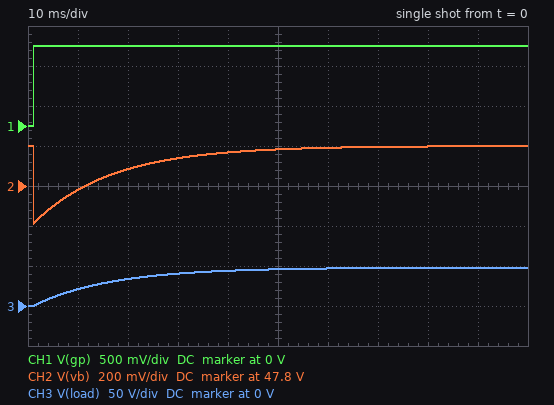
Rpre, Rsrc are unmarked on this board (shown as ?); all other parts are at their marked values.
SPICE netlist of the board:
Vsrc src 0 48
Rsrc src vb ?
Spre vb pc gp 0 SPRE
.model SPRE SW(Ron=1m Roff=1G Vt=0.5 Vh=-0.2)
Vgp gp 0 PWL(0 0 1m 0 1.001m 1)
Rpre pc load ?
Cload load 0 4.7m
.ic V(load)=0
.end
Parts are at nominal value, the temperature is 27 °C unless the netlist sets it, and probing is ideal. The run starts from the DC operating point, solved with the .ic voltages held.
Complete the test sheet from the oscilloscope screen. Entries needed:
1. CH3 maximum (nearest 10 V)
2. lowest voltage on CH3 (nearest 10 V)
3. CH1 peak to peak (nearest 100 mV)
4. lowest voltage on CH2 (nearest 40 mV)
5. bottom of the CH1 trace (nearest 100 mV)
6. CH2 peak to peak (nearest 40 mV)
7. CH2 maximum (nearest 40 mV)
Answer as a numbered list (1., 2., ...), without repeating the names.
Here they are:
1. 50 V
2. 0 V
3. 1.0 V
4. 47.60 V
5. 0 V
6. 400 mV
7. 48.00 V
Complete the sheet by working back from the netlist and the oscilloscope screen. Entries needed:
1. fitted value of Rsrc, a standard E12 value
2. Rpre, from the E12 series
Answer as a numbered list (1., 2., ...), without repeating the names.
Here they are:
1. 0.027 Ω
2. 3.3 Ω
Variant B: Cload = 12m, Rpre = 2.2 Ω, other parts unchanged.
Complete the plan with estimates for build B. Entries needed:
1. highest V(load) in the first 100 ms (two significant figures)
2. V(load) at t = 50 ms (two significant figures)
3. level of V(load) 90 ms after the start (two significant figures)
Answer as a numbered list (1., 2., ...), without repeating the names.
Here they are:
1. 47 V
2. 40 V
3. 46 V
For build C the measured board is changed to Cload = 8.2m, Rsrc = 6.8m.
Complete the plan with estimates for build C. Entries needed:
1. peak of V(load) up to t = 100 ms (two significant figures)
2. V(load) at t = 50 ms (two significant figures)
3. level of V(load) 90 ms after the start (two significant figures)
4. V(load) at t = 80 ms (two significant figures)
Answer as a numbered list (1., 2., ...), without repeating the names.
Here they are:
1. 47 V
2. 40 V
3. 46 V
4. 45 V
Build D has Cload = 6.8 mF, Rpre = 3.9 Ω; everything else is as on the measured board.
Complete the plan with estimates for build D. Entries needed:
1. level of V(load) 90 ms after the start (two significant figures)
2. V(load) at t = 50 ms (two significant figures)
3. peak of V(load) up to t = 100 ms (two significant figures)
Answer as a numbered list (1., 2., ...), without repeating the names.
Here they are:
1. 46 V
2. 40 V
3. 47 V
